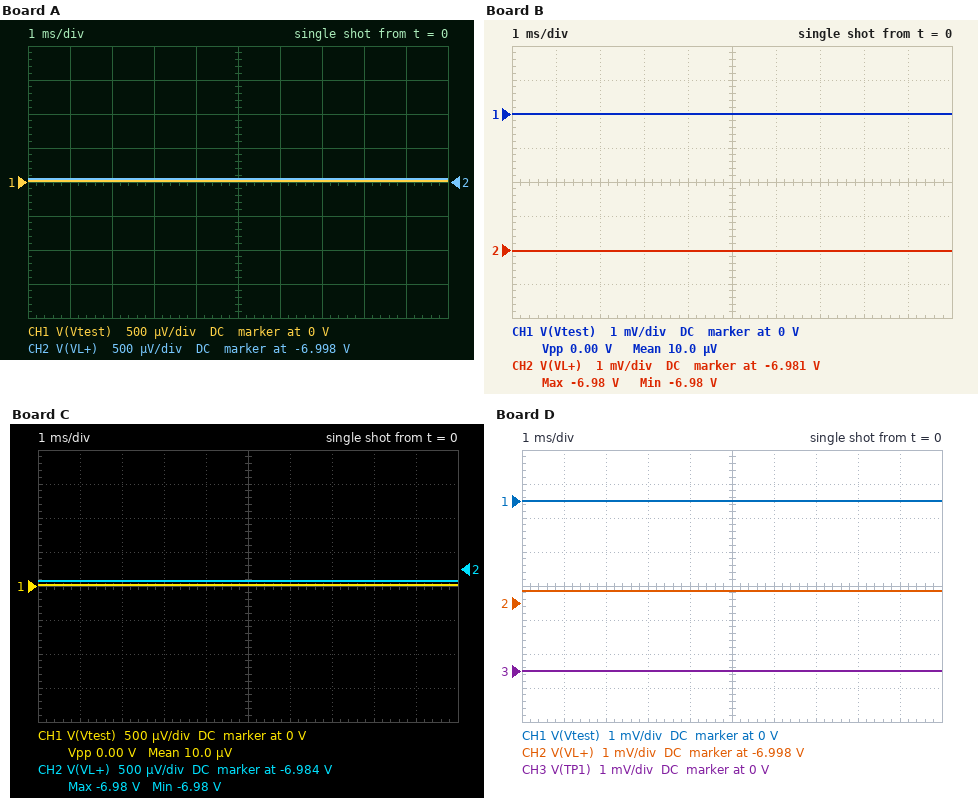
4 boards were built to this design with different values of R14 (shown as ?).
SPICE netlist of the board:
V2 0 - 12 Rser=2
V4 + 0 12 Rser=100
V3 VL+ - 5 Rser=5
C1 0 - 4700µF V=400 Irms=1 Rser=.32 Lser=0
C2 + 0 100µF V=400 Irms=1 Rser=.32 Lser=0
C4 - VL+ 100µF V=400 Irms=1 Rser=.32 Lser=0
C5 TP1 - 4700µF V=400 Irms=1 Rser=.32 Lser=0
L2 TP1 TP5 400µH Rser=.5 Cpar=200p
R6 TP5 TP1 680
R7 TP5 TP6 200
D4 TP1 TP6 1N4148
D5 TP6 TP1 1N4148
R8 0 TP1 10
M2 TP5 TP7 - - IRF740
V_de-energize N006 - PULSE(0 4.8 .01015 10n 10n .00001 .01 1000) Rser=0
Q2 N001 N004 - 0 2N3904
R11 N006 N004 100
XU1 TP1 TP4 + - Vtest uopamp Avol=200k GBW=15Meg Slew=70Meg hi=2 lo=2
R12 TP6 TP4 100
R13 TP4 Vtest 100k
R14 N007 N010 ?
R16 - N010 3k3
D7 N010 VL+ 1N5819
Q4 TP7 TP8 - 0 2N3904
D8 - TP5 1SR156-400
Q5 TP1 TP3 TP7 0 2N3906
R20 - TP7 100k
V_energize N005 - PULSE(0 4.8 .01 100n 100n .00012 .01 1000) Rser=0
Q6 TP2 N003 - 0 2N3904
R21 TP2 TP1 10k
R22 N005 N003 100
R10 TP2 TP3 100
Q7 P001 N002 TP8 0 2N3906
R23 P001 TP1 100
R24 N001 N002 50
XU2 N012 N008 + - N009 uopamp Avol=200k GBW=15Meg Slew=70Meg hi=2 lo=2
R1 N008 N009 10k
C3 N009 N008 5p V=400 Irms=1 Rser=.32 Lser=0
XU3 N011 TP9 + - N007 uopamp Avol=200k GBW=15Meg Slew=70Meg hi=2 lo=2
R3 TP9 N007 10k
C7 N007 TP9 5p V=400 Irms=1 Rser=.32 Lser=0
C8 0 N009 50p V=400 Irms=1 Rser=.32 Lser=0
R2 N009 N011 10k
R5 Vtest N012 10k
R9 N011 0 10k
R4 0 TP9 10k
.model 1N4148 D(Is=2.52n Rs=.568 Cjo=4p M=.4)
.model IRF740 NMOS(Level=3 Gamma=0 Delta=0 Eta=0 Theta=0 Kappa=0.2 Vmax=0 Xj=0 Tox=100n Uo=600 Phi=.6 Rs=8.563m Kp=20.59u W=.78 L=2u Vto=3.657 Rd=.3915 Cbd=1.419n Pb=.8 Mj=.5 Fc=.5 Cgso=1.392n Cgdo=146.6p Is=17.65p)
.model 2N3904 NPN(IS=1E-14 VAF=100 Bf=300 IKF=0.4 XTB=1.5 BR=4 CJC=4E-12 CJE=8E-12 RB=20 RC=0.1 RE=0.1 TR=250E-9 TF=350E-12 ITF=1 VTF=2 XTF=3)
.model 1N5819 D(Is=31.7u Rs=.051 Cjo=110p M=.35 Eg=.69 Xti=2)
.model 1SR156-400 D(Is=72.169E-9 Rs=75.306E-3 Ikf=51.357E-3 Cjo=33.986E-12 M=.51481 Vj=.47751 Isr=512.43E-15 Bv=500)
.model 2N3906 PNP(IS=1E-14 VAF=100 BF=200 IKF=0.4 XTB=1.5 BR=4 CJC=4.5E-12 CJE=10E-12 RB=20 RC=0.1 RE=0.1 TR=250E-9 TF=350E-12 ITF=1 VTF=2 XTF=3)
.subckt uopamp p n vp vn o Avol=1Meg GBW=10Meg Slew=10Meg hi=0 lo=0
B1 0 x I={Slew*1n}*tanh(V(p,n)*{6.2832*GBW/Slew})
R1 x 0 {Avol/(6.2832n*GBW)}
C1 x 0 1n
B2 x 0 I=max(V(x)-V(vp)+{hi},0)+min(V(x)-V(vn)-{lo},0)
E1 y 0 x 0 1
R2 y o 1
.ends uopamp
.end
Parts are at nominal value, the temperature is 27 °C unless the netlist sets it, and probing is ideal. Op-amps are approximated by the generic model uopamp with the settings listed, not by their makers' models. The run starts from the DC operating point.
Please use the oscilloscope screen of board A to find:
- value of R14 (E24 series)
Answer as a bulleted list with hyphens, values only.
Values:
- 7.5 kΩ
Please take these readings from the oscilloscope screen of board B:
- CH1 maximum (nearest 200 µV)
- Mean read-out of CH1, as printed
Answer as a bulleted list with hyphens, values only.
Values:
- 0 V
- 10.0 µV
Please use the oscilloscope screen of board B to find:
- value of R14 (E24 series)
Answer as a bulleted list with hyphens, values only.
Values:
- 1.8 kΩ
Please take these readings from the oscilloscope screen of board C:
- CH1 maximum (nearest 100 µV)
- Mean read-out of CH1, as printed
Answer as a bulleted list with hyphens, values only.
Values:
- 0 V
- 10.0 µV
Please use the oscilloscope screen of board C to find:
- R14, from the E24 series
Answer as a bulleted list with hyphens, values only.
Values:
- 2 kΩ
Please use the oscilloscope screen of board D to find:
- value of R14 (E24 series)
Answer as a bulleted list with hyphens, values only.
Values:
- 6.2 kΩ
